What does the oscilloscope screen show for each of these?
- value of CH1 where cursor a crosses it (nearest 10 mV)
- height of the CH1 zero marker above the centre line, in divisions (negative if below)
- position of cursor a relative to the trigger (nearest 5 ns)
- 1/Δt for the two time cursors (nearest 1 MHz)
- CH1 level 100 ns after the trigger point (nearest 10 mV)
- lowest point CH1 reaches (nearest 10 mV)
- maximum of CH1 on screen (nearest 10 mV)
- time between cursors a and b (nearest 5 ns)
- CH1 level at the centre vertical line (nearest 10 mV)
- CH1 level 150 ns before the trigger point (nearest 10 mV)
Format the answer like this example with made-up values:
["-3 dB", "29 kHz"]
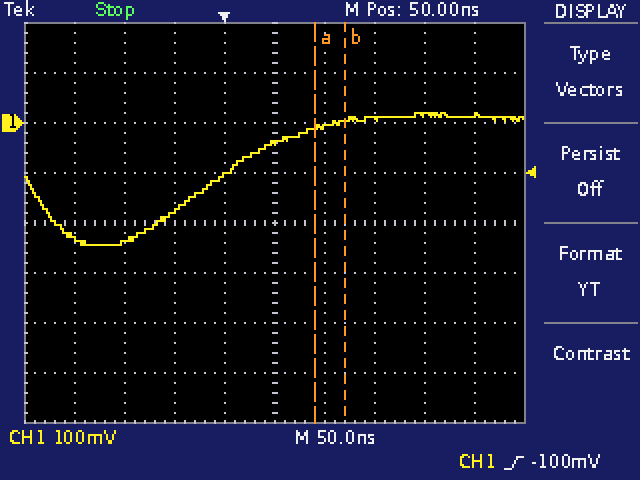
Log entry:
["-10 mV", "+2.0 div", "+90 ns", "33 MHz", "-10 mV", "-240 mV", "20 mV", "30 ns", "-40 mV", "-230 mV"]
